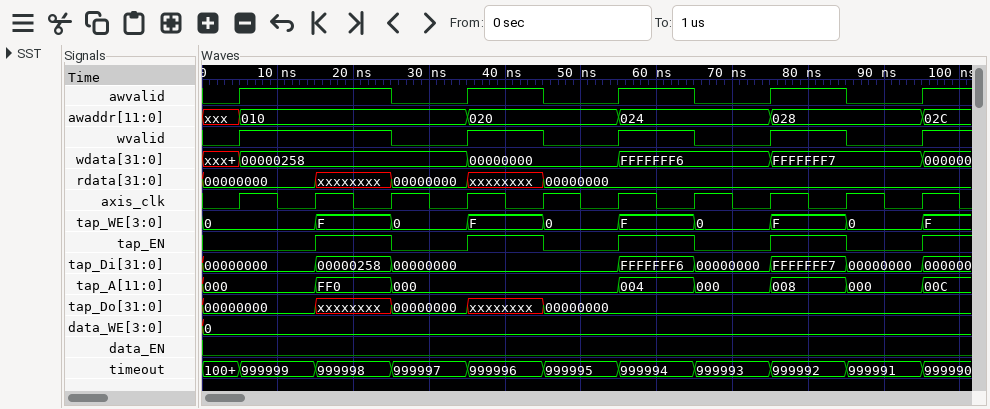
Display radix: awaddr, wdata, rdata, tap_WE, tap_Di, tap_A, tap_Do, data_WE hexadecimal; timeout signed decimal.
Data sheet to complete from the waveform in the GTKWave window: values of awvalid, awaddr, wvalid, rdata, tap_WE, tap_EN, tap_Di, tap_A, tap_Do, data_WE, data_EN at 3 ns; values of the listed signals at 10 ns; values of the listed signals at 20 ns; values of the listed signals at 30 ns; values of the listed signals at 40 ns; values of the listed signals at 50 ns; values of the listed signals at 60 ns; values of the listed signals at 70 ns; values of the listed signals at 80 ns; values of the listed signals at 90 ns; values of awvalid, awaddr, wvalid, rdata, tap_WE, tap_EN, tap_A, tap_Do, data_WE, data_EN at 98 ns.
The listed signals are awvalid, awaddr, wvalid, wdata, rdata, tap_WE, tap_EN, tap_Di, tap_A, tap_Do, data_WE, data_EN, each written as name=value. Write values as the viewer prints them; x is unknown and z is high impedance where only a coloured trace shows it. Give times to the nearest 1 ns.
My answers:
awvalid=0, awaddr=xxx, wvalid=0, rdata=00000000, tap_WE=0, tap_EN=0, tap_Di=00000000, tap_A=000, tap_Do=00000000, data_WE=0, data_EN=0
awvalid=1, awaddr=010, wvalid=1, wdata=00000258, rdata=00000000, tap_WE=0, tap_EN=0, tap_Di=00000000, tap_A=000, tap_Do=00000000, data_WE=0, data_EN=0
awvalid=1, awaddr=010, wvalid=1, wdata=00000258, rdata=xxxxxxxx, tap_WE=F, tap_EN=1, tap_Di=00000258, tap_A=FF0, tap_Do=xxxxxxxx, data_WE=0, data_EN=0
awvalid=0, awaddr=010, wvalid=0, wdata=00000258, rdata=00000000, tap_WE=0, tap_EN=0, tap_Di=00000000, tap_A=000, tap_Do=00000000, data_WE=0, data_EN=0
awvalid=1, awaddr=020, wvalid=1, wdata=00000000, rdata=xxxxxxxx, tap_WE=F, tap_EN=1, tap_Di=00000000, tap_A=000, tap_Do=xxxxxxxx, data_WE=0, data_EN=0
awvalid=0, awaddr=020, wvalid=0, wdata=00000000, rdata=00000000, tap_WE=0, tap_EN=0, tap_Di=00000000, tap_A=000, tap_Do=00000000, data_WE=0, data_EN=0
awvalid=1, awaddr=024, wvalid=1, wdata=FFFFFFF6, rdata=00000000, tap_WE=F, tap_EN=1, tap_Di=FFFFFFF6, tap_A=004, tap_Do=00000000, data_WE=0, data_EN=0
awvalid=0, awaddr=024, wvalid=0, wdata=FFFFFFF6, rdata=00000000, tap_WE=0, tap_EN=0, tap_Di=00000000, tap_A=000, tap_Do=00000000, data_WE=0, data_EN=0
awvalid=1, awaddr=028, wvalid=1, wdata=FFFFFFF7, rdata=00000000, tap_WE=F, tap_EN=1, tap_Di=FFFFFFF7, tap_A=008, tap_Do=00000000, data_WE=0, data_EN=0
awvalid=0, awaddr=028, wvalid=0, wdata=FFFFFFF7, rdata=00000000, tap_WE=0, tap_EN=0, tap_Di=00000000, tap_A=000, tap_Do=00000000, data_WE=0, data_EN=0
awvalid=1, awaddr=02C, wvalid=1, rdata=00000000, tap_WE=F, tap_EN=1, tap_A=00C, tap_Do=00000000, data_WE=0, data_EN=0
